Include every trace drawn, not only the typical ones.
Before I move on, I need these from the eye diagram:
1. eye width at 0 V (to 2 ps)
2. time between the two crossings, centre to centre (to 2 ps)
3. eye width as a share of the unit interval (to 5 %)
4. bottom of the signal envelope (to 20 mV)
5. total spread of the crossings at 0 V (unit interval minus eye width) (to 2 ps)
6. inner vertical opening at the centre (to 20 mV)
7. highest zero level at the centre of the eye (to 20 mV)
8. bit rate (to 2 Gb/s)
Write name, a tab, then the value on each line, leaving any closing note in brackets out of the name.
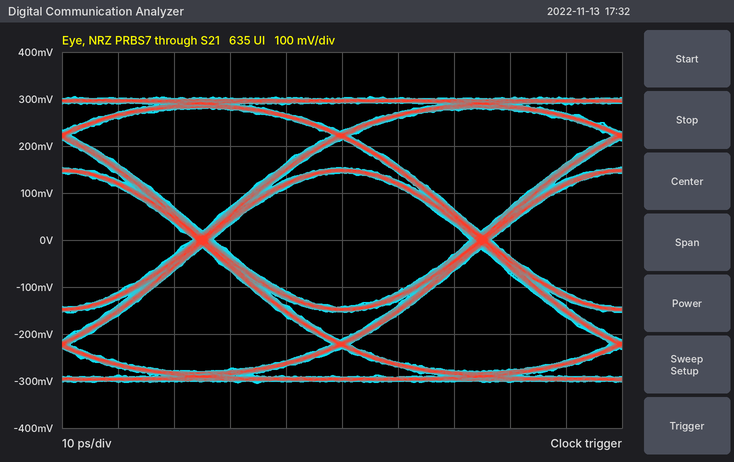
eye width at 0 V	46 ps
time between the two crossings, centre to centre	50 ps
eye width as a share of the unit interval	90 %
bottom of the signal envelope	-300 mV
total spread of the crossings at 0 V (unit interval minus eye width)	4 ps
inner vertical opening at the centre	280 mV
highest zero level at the centre of the eye	-140 mV
bit rate	20 Gb/s
